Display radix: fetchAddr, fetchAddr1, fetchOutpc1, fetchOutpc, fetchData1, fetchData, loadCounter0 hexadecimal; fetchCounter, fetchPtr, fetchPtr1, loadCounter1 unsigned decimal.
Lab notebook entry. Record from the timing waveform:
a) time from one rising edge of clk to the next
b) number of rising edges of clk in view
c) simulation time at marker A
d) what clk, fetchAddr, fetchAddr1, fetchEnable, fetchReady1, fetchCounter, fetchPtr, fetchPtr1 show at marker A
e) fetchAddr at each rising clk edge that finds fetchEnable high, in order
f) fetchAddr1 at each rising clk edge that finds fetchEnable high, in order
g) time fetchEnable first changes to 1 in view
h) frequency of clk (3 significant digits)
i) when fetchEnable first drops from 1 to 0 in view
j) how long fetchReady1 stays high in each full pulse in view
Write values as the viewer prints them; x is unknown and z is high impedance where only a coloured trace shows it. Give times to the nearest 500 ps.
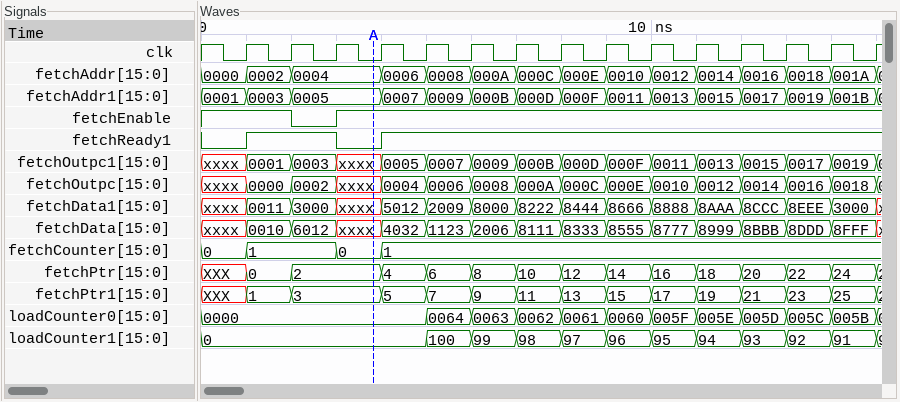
1000 ps
15
4000 ps
clk=0, fetchAddr=0004, fetchAddr1=0005, fetchEnable=1, fetchReady1=0, fetchCounter=0, fetchPtr=2, fetchPtr1=3
0000, 0002, 0004, 0006, 0008, 000A, 000C, 000E, 0010, 0012, 0014, 0016, 0018, 001A
0001, 0003, 0005, 0007, 0009, 000B, 000D, 000F, 0011, 0013, 0015, 0017, 0019, 001B
3000 ps
1.00 GHz
2000 ps
2000 ps
